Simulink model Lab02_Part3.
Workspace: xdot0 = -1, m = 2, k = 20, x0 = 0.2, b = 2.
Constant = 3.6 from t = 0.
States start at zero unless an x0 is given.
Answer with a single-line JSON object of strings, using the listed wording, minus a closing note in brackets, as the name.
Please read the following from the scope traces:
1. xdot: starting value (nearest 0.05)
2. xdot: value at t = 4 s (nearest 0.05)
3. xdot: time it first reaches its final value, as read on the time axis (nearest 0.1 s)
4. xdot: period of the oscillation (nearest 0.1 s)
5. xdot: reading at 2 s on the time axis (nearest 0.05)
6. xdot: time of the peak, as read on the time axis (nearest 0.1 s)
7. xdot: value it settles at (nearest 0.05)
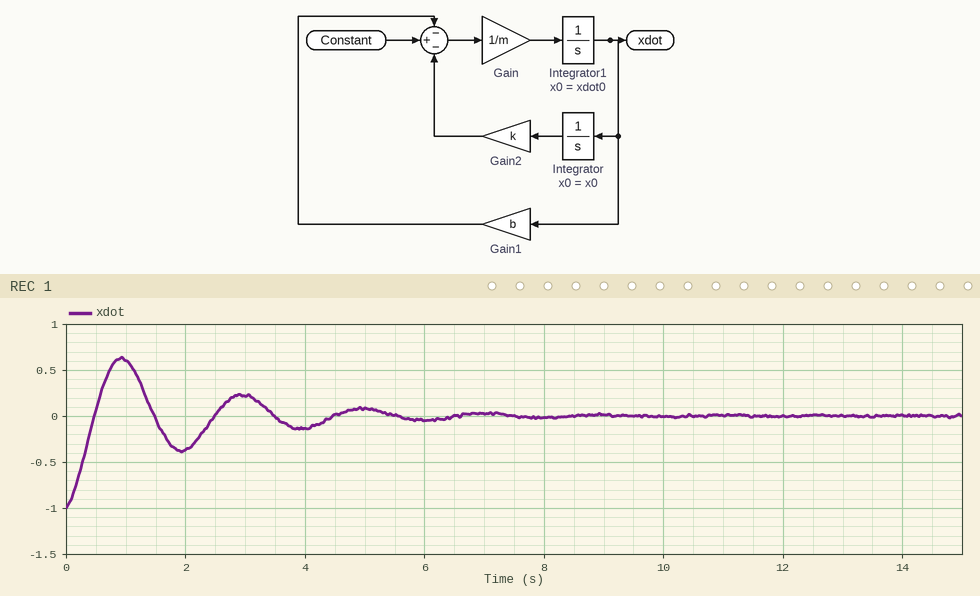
{"xdot: starting value": "-1.00", "xdot: value at t = 4 s": "-0.15", "xdot: time it first reaches its final value, as read on the time axis": "0.5 s", "xdot: period of the oscillation": "2.0 s", "xdot: reading at 2 s on the time axis": "-0.35", "xdot: time of the peak, as read on the time axis": "0.9 s", "xdot: value it settles at": "0.00"}
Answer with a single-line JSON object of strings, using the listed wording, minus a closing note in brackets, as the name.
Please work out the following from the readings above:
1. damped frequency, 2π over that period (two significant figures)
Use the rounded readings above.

{"damped frequency, 2π over that period": "3.1 rad/s"}
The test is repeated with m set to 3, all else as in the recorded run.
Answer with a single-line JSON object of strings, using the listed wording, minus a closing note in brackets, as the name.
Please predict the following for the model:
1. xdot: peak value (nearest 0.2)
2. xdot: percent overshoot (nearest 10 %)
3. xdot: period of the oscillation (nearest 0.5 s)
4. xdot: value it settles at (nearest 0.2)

{"xdot: peak value": "0.6", "xdot: percent overshoot": "70 %", "xdot: period of the oscillation": "2.5 s", "xdot: value it settles at": "0.0"}
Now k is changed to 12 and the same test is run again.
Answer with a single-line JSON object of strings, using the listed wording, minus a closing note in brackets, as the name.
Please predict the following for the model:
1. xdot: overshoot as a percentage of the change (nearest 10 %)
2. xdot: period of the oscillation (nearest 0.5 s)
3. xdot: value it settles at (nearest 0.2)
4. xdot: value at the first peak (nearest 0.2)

{"xdot: overshoot as a percentage of the change": "60 %", "xdot: period of the oscillation": "2.5 s", "xdot: value it settles at": "0.0", "xdot: value at the first peak": "0.6"}
